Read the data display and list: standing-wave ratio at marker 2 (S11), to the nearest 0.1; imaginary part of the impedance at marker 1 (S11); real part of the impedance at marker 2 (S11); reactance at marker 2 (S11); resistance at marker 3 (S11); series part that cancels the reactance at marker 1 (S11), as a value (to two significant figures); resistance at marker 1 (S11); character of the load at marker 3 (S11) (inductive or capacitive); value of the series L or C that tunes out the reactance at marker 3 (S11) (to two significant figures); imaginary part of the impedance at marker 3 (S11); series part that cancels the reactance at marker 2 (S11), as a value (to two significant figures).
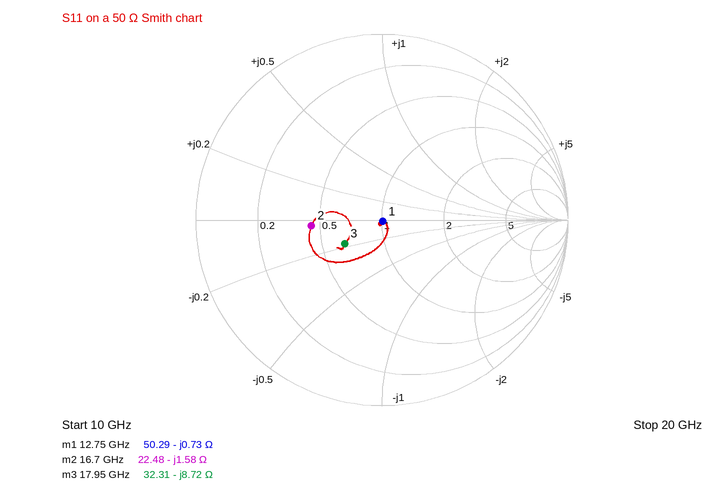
2.2
-0.73 Ω
22.48 Ω
-1.58 Ω
32.31 Ω
9.1 pH
50.29 Ω
capacitive
77 pH
-8.72 Ω
15 pH
